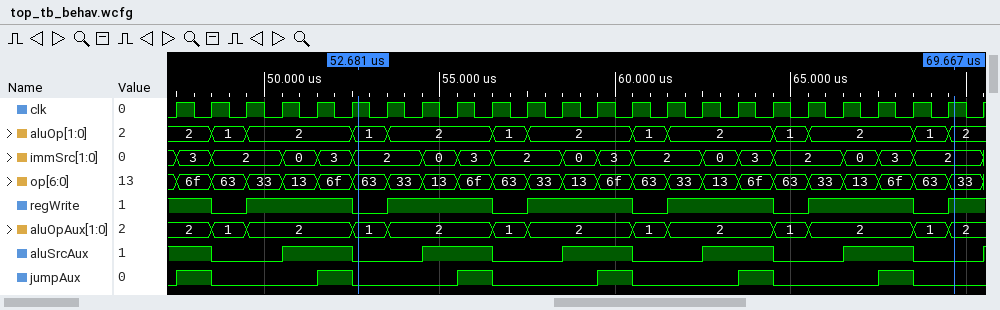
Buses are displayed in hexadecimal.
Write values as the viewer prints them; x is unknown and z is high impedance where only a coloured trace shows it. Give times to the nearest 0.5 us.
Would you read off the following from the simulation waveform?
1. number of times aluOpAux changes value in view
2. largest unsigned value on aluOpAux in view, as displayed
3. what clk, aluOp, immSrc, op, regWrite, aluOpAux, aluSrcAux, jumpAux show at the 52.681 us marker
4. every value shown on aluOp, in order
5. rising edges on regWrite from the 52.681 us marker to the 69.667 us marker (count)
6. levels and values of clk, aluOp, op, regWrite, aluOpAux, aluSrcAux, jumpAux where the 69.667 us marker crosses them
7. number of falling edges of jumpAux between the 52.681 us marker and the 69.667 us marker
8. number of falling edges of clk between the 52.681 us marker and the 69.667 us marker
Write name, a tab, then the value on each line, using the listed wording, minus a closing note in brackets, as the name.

number of times aluOpAux changes value in view	12
largest unsigned value on aluOpAux in view, as displayed	2
what clk, aluOp, immSrc, op, regWrite, aluOpAux, aluSrcAux, jumpAux show at the 52.681 us marker	clk=1, aluOp=1, immSrc=2, op=63, regWrite=0, aluOpAux=1, aluSrcAux=0, jumpAux=0
every value shown on aluOp, in order	2, 1, 2, 1, 2, 1, 2, 1, 2, 1, 2, 1, 2
rising edges on regWrite from the 52.681 us marker to the 69.667 us marker	5
levels and values of clk, aluOp, op, regWrite, aluOpAux, aluSrcAux, jumpAux where the 69.667 us marker crosses them	clk=1, aluOp=2, op=33, regWrite=1, aluOpAux=2, aluSrcAux=0, jumpAux=0
number of falling edges of jumpAux between the 52.681 us marker and the 69.667 us marker	4
number of falling edges of clk between the 52.681 us marker and the 69.667 us marker	17
